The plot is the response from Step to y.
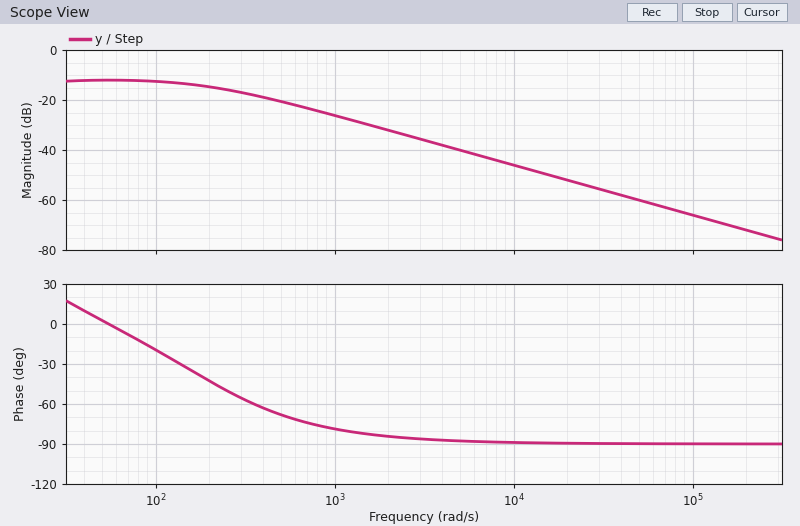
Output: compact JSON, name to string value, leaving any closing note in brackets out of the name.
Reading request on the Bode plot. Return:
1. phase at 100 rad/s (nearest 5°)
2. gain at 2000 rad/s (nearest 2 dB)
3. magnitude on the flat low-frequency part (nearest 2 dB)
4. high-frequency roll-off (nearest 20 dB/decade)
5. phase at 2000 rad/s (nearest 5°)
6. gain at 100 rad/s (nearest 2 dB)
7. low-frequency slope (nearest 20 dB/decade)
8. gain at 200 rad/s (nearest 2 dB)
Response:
{"phase at 100 rad/s": "-20°", "gain at 2000 rad/s": "-32 dB", "magnitude on the flat low-frequency part": "-12 dB", "high-frequency roll-off": "-20 dB/decade", "phase at 2000 rad/s": "-85°", "gain at 100 rad/s": "-12 dB", "low-frequency slope": "0 dB/decade", "gain at 200 rad/s": "-14 dB"}
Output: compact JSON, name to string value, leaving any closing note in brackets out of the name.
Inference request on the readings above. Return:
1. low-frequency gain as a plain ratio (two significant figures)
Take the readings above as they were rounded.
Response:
{"low-frequency gain as a plain ratio": "0.25"}
